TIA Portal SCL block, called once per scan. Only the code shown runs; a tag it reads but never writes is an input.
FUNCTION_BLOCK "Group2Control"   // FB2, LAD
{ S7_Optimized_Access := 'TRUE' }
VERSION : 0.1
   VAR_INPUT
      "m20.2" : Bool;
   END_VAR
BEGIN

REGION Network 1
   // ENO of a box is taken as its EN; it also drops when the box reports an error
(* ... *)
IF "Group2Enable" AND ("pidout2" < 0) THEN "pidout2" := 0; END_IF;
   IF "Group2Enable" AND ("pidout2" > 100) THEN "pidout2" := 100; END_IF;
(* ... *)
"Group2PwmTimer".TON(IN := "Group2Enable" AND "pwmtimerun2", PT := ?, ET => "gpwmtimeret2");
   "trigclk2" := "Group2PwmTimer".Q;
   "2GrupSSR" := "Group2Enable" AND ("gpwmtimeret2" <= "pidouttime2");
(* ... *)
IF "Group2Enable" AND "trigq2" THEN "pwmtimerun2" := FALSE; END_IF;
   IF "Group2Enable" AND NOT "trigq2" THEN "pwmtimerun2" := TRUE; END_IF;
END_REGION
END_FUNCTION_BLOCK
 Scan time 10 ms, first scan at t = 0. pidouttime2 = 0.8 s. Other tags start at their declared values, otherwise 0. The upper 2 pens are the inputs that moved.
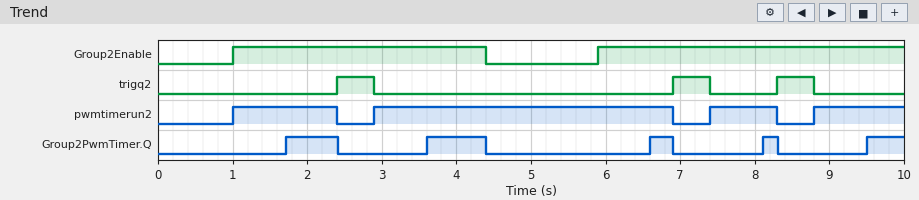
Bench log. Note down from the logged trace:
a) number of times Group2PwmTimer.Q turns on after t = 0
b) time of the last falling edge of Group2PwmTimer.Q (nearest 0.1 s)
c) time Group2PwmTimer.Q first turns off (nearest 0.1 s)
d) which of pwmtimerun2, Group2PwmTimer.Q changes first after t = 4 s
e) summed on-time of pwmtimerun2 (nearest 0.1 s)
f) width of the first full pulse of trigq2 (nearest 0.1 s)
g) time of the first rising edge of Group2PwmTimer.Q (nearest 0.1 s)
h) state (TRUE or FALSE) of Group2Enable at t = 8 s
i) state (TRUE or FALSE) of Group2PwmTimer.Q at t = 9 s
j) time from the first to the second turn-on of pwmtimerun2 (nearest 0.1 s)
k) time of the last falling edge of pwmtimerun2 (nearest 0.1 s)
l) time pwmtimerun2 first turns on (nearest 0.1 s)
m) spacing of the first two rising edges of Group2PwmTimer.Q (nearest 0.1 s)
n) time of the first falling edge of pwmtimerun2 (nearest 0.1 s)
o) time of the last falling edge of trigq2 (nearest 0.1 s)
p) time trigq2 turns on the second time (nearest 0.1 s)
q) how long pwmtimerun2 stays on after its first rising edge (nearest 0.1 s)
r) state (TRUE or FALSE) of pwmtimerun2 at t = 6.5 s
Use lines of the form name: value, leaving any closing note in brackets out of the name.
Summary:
number of times Group2PwmTimer.Q turns on after t = 0: 5
time of the last falling edge of Group2PwmTimer.Q: 8.3 s
time Group2PwmTimer.Q first turns off: 2.4 s
which of pwmtimerun2, Group2PwmTimer.Q changes first after t = 4 s: Group2PwmTimer.Q
summed on-time of pwmtimerun2: 7.5 s
width of the first full pulse of trigq2: 0.5 s
time of the first rising edge of Group2PwmTimer.Q: 1.7 s
state (TRUE or FALSE) of Group2Enable at t = 8 s: TRUE
state (TRUE or FALSE) of Group2PwmTimer.Q at t = 9 s: FALSE
time from the first to the second turn-on of pwmtimerun2: 1.9 s
time of the last falling edge of pwmtimerun2: 8.3 s
time pwmtimerun2 first turns on: 1.0 s
spacing of the first two rising edges of Group2PwmTimer.Q: 1.9 s
time of the first falling edge of pwmtimerun2: 2.4 s
time of the last falling edge of trigq2: 8.8 s
time trigq2 turns on the second time: 6.9 s
how long pwmtimerun2 stays on after its first rising edge: 1.4 s
state (TRUE or FALSE) of pwmtimerun2 at t = 6.5 s: TRUE
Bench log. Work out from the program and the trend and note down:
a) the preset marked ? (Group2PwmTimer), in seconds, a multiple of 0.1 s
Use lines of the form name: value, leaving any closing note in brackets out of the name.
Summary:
the preset marked ? (Group2PwmTimer), in seconds, a multiple of 0.1 s: 0.7 s
